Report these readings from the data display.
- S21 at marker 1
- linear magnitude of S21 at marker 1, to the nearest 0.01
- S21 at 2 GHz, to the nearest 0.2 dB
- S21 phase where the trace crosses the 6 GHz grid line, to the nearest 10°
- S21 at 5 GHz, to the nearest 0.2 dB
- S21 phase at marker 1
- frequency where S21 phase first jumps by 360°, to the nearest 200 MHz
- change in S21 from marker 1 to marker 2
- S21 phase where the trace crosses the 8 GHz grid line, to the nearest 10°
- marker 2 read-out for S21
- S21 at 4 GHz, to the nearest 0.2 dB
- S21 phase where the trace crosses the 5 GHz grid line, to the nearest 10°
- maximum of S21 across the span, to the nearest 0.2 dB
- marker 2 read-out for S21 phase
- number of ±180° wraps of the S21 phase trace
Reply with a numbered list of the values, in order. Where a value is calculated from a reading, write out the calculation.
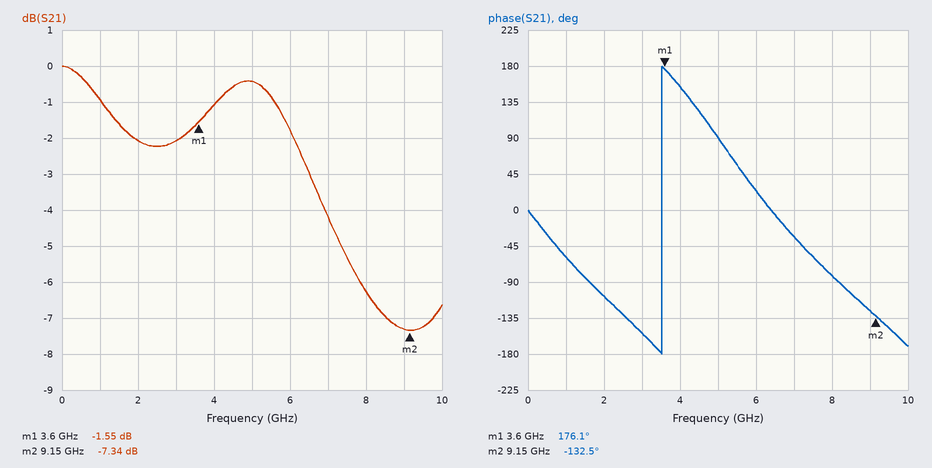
1. -1.55 dB
2. 10^(-1.55/20) ≈ 0.84
3. -2.0 dB
4. 20°
5. -0.4 dB
6. 176.1°
7. 3.6 GHz
8. -7.34 − (-1.55) = -5.79 dB
9. -80°
10. -7.34 dB
11. -1.0 dB
12. 90°
13. 0.0 dB
14. -132.5°
15. 1
